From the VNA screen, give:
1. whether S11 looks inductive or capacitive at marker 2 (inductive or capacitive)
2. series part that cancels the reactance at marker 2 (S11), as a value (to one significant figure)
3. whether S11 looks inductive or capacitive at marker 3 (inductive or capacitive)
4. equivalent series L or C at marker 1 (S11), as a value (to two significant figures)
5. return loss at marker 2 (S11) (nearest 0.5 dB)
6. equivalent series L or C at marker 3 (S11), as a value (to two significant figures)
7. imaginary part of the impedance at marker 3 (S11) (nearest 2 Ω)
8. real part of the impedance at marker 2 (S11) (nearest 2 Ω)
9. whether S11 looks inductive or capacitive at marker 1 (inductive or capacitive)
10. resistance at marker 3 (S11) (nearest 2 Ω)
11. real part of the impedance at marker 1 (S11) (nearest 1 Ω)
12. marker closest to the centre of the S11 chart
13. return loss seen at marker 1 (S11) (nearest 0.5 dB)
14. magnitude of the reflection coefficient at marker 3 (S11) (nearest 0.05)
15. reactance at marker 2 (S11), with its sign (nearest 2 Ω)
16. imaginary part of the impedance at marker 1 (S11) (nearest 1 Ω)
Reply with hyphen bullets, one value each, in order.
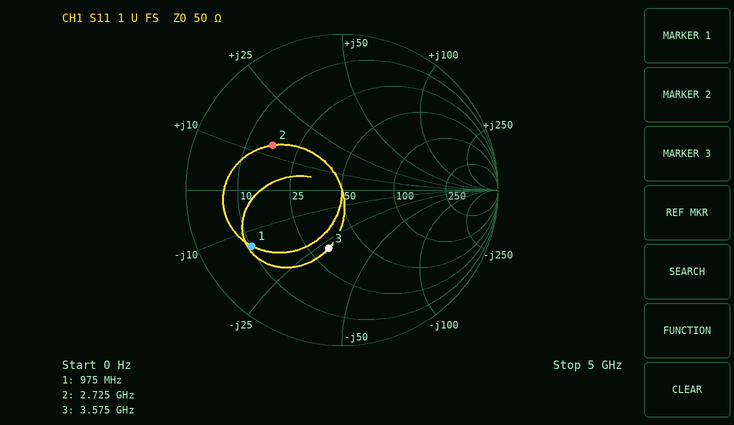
- inductive
- 4 pF
- capacitive
- 12 pF
- 5.5 dB
- 1.6 pF
- -28 Ω
- 16 Ω
- capacitive
- 32 Ω
- 10 Ω
- marker 3
- 3.5 dB
- 0.40
- +14 Ω
- -14 Ω
